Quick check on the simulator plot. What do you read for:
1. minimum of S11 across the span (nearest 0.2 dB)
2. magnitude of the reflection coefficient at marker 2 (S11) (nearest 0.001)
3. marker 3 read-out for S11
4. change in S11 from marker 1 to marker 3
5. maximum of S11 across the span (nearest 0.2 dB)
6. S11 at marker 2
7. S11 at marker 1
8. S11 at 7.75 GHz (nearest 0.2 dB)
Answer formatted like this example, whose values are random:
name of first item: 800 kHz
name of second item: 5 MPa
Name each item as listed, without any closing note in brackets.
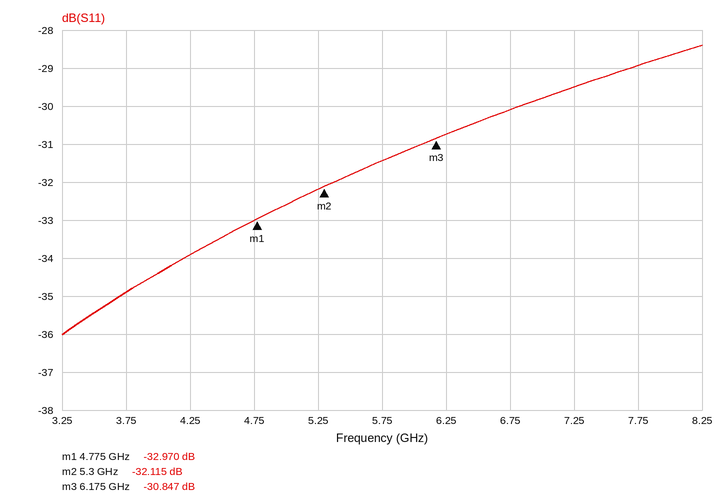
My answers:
minimum of S11 across the span: -36.0 dB
magnitude of the reflection coefficient at marker 2 (S11): 0.025
marker 3 read-out for S11: -30.847 dB
change in S11 from marker 1 to marker 3: 2.123 dB
maximum of S11 across the span: -28.4 dB
S11 at marker 2: -32.115 dB
S11 at marker 1: -32.970 dB
S11 at 7.75 GHz: -29.0 dB
